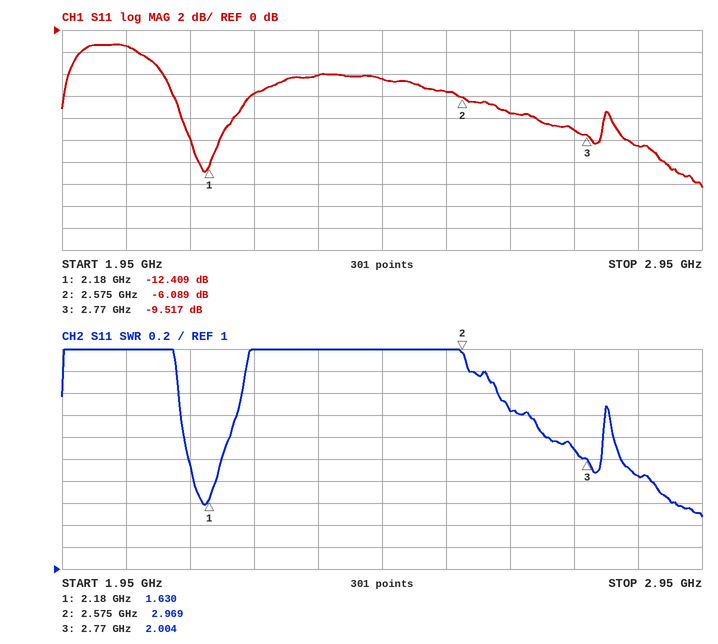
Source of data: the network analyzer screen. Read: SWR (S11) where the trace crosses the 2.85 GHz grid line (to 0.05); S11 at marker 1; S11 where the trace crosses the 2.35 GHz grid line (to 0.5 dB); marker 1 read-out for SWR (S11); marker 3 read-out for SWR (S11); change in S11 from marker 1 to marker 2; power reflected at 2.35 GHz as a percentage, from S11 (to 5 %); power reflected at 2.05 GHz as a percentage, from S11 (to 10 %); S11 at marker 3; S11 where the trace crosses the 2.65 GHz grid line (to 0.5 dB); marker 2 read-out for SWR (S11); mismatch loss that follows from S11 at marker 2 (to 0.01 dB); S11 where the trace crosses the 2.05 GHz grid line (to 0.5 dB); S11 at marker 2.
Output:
1.85
-12.409 dB
-4.0 dB
1.630
2.004
6.320 dB
40 %
70 %
-9.517 dB
-7.5 dB
2.969
1.23 dB
-1.5 dB
-6.089 dB
